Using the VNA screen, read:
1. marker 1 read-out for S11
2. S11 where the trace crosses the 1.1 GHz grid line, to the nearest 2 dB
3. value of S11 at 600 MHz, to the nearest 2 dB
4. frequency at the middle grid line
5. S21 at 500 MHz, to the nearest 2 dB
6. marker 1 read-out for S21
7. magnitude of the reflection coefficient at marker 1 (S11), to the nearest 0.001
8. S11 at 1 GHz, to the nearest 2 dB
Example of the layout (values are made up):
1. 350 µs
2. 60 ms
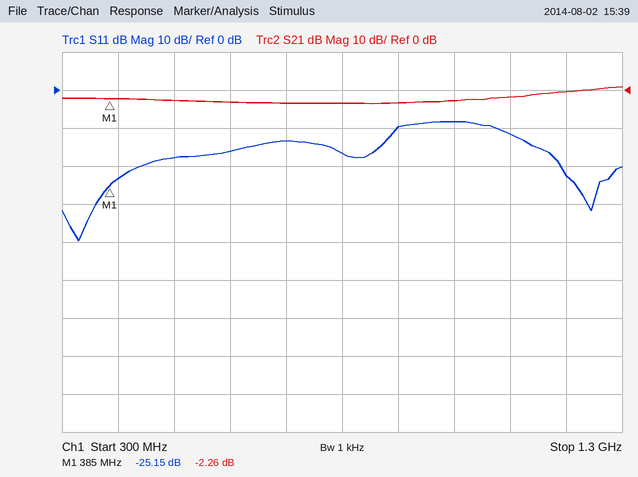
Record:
1. -25.15 dB
2. -12 dB
3. -16 dB
4. 800 MHz
5. -2 dB
6. -2.26 dB
7. 0.055
8. -8 dB
